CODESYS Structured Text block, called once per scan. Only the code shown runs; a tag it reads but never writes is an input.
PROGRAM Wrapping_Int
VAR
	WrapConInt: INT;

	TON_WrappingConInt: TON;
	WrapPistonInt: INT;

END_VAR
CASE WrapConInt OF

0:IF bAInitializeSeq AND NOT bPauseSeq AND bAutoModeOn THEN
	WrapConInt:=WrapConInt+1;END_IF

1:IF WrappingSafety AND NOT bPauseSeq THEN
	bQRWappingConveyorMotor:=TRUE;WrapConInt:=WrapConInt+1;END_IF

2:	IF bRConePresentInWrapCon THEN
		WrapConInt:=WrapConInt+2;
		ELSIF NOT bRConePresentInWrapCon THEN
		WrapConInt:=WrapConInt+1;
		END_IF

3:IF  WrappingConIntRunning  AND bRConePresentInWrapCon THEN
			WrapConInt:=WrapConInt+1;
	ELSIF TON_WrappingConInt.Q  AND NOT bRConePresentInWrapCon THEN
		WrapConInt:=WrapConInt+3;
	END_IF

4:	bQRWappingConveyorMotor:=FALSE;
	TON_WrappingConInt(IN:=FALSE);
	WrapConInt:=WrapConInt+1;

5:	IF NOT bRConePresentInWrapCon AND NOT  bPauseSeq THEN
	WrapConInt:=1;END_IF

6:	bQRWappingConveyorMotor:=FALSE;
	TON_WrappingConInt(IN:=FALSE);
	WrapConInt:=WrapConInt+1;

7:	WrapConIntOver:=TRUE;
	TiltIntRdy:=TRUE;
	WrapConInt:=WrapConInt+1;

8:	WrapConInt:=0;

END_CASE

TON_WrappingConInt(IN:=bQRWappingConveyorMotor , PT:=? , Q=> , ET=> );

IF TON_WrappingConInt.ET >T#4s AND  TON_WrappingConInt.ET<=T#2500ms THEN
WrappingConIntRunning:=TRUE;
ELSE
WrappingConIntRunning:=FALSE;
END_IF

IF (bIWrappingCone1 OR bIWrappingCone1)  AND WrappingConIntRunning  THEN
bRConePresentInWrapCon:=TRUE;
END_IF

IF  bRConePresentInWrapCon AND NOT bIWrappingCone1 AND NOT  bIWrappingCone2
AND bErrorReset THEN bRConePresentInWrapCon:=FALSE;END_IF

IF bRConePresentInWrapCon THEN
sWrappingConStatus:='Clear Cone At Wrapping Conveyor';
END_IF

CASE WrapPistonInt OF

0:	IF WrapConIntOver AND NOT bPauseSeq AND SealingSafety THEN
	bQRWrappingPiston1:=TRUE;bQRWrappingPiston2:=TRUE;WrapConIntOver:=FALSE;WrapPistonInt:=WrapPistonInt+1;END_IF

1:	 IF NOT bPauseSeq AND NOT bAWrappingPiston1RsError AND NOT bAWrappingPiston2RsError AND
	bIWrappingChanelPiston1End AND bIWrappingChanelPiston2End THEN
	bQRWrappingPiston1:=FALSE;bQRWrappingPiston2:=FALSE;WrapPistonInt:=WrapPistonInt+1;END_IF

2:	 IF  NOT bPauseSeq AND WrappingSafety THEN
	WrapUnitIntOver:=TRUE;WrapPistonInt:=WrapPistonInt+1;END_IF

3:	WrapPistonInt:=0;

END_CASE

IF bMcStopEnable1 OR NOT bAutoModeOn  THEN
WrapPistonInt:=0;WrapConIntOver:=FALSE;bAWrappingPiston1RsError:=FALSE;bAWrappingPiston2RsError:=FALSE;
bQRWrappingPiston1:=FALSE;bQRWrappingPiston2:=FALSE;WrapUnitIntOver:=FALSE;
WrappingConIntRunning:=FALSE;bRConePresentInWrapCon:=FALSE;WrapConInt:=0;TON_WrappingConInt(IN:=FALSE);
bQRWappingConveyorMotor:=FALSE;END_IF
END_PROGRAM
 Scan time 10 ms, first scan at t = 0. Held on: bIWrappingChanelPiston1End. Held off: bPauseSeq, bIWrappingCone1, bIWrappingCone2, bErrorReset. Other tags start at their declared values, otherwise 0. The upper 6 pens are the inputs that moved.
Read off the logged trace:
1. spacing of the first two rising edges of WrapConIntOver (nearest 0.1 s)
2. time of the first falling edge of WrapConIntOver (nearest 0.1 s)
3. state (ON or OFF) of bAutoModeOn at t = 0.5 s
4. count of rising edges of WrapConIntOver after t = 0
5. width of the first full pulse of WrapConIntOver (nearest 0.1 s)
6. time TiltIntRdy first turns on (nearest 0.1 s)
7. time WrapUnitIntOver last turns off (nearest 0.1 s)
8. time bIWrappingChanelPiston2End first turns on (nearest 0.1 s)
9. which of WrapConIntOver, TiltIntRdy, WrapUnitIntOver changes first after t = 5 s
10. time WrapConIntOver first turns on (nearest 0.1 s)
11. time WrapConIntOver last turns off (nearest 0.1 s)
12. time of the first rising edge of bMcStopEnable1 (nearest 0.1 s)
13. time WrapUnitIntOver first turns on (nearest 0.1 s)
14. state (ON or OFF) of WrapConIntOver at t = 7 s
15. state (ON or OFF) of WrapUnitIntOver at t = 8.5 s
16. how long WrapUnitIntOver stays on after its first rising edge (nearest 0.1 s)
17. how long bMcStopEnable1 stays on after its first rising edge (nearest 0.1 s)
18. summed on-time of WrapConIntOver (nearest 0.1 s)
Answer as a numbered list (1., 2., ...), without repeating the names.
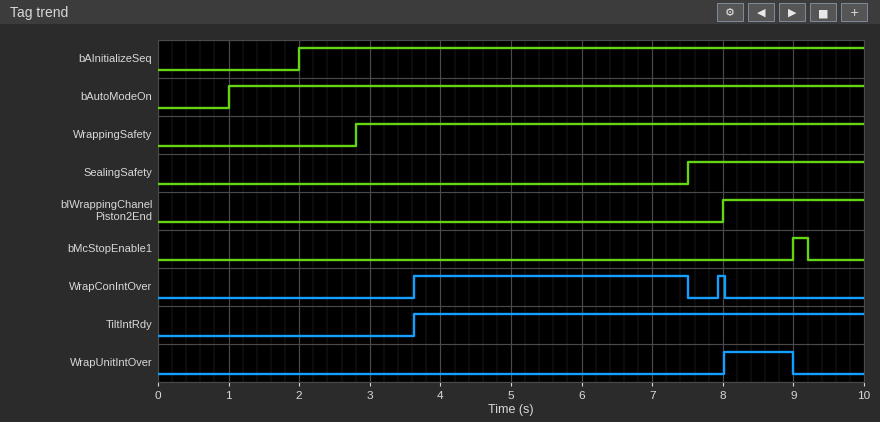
1. 4.3 s
2. 7.5 s
3. OFF
4. 2
5. 3.9 s
6. 3.6 s
7. 9.0 s
8. 8.0 s
9. WrapConIntOver
10. 3.6 s
11. 8.0 s
12. 9.0 s
13. 8.0 s
14. ON
15. ON
16. 1.0 s
17. 0.2 s
18. 4.0 s
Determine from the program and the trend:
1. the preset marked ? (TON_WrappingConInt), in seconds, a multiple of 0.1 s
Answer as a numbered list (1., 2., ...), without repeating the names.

1. 0.8 s
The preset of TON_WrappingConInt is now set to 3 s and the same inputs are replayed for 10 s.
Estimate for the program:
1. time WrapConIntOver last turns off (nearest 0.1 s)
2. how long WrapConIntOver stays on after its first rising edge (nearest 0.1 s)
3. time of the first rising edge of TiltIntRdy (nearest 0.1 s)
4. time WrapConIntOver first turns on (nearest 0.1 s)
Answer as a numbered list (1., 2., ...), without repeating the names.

1. 7.5 s
2. 1.7 s
3. 5.8 s
4. 5.8 s
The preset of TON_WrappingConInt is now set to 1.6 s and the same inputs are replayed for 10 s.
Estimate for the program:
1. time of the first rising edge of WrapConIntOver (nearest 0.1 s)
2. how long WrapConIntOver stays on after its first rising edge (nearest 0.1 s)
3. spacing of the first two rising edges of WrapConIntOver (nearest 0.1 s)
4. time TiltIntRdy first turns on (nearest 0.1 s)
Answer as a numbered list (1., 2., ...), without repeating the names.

1. 4.4 s
2. 3.1 s
3. 3.3 s
4. 4.4 s
